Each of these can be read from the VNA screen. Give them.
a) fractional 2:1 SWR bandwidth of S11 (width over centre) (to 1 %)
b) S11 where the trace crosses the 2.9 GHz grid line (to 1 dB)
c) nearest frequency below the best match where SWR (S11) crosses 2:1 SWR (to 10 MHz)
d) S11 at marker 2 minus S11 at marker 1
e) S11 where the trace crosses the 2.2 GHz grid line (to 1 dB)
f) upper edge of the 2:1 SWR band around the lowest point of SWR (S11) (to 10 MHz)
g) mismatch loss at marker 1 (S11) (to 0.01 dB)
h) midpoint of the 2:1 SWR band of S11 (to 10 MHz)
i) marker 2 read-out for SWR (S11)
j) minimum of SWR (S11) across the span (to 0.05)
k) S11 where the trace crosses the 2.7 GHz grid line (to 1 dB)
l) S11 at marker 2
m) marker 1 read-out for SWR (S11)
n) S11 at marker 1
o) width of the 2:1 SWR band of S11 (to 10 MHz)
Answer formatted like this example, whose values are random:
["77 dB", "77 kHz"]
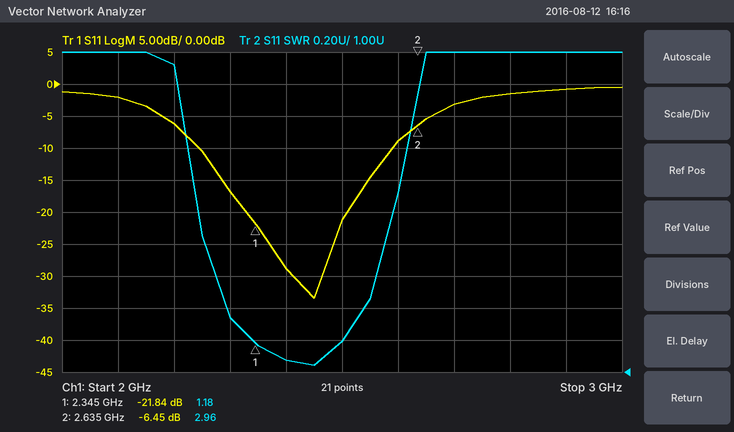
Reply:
["14 %", "-1 dB", "2.24 GHz", "15.39 dB", "-6 dB", "2.59 GHz", "0.03 dB", "2.42 GHz", "2.96", "1.05", "-3 dB", "-6.45 dB", "1.18", "-21.84 dB", "350 MHz"]
